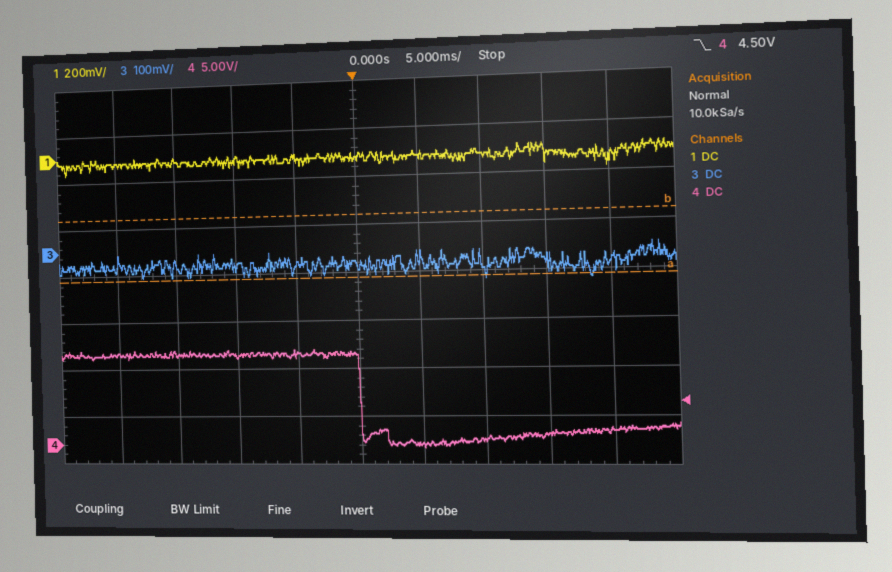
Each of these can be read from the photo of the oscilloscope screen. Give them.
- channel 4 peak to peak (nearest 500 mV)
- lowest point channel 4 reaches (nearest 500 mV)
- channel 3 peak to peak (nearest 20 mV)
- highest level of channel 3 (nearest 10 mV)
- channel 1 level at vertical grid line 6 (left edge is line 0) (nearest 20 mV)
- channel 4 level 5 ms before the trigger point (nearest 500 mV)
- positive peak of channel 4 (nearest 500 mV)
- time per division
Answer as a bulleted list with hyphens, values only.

- 10.0 V
- 0.0 V
- 60 mV
- 0 mV
- -20 mV
- 9.5 V
- 10.0 V
- 5 ms
